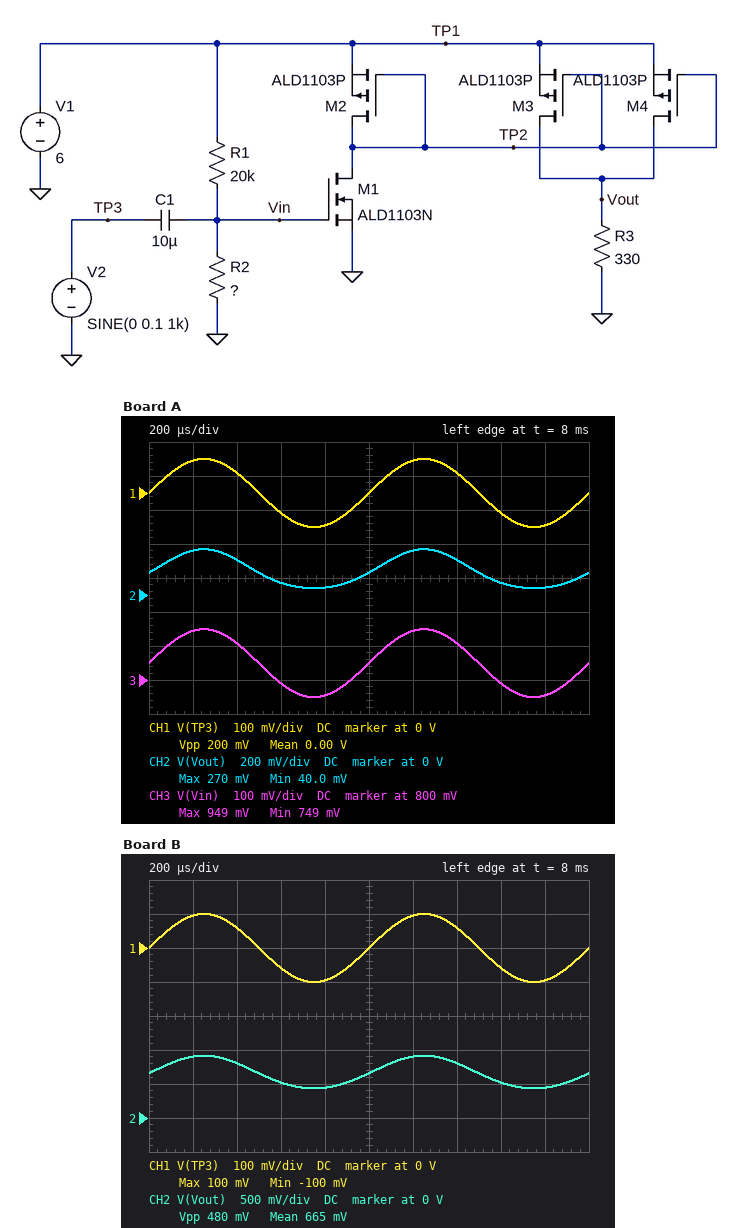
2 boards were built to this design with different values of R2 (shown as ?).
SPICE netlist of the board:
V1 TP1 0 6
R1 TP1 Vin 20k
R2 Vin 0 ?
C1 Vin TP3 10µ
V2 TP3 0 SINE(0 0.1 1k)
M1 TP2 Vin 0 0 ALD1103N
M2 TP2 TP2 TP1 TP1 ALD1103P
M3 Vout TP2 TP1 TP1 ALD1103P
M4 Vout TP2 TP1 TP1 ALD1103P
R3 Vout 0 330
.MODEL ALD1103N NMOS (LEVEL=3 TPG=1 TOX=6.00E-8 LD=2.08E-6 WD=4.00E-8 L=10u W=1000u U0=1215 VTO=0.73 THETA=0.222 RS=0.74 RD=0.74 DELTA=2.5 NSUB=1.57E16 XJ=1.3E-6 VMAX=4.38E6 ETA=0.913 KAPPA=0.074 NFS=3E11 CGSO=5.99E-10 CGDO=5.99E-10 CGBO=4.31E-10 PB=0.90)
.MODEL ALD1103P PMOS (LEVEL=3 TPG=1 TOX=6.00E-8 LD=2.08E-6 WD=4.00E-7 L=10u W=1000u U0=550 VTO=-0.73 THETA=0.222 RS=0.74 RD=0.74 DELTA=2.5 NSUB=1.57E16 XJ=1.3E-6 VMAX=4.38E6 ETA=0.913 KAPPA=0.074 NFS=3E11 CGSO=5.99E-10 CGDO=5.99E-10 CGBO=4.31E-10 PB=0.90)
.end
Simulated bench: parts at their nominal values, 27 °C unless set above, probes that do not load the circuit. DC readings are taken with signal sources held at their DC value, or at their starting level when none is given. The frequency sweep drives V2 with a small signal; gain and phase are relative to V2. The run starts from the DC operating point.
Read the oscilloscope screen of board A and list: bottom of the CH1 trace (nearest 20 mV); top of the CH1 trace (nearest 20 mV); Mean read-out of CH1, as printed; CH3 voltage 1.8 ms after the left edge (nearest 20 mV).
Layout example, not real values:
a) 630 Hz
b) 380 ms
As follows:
a) -100 mV
b) 100 mV
c) 0.00 V
d) 760 mV
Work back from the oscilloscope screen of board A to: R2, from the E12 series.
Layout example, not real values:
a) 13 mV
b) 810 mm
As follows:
a) 3.3 kΩ
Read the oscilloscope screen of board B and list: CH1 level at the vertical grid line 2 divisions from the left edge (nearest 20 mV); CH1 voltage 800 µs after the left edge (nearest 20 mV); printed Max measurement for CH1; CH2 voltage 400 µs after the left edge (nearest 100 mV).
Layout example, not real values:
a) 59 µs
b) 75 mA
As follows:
a) 60 mV
b) -100 mV
c) 100 mV
d) 800 mV
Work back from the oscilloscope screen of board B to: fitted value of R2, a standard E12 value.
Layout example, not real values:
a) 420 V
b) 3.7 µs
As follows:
a) 4.7 kΩ
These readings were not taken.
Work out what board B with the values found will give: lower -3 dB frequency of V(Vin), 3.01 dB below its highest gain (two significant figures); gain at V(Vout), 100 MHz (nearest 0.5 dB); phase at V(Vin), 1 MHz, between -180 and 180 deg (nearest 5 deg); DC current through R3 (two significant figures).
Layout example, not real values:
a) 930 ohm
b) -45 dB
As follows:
a) 4.2 Hz
b) -3.0 dB
c) 0 deg
d) 2.0 mA
